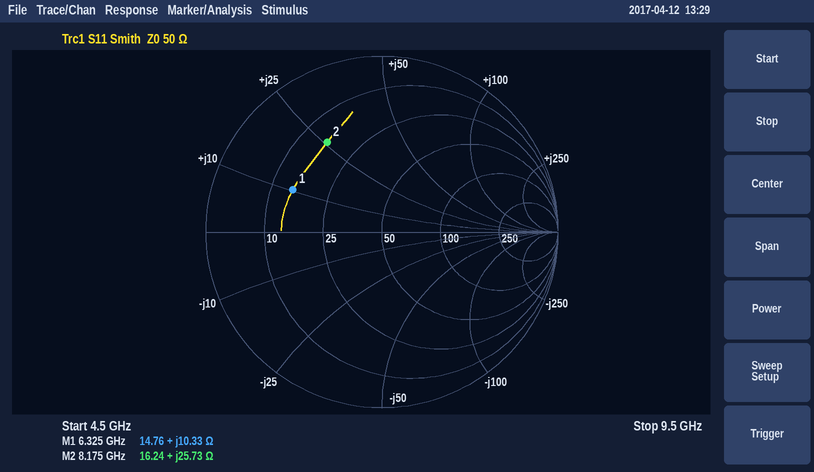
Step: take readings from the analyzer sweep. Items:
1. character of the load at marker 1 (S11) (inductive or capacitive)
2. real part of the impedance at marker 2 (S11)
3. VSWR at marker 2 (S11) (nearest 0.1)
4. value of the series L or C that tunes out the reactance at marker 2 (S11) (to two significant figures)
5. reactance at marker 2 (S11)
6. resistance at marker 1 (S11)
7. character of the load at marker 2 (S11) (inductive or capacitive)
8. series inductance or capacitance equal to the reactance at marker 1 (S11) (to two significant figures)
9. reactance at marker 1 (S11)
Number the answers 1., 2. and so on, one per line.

1. inductive
2. 16.24 Ω
3. 4.0
4. 760 fF
5. +25.73 Ω
6. 14.76 Ω
7. inductive
8. 260 pH
9. +10.33 Ω
